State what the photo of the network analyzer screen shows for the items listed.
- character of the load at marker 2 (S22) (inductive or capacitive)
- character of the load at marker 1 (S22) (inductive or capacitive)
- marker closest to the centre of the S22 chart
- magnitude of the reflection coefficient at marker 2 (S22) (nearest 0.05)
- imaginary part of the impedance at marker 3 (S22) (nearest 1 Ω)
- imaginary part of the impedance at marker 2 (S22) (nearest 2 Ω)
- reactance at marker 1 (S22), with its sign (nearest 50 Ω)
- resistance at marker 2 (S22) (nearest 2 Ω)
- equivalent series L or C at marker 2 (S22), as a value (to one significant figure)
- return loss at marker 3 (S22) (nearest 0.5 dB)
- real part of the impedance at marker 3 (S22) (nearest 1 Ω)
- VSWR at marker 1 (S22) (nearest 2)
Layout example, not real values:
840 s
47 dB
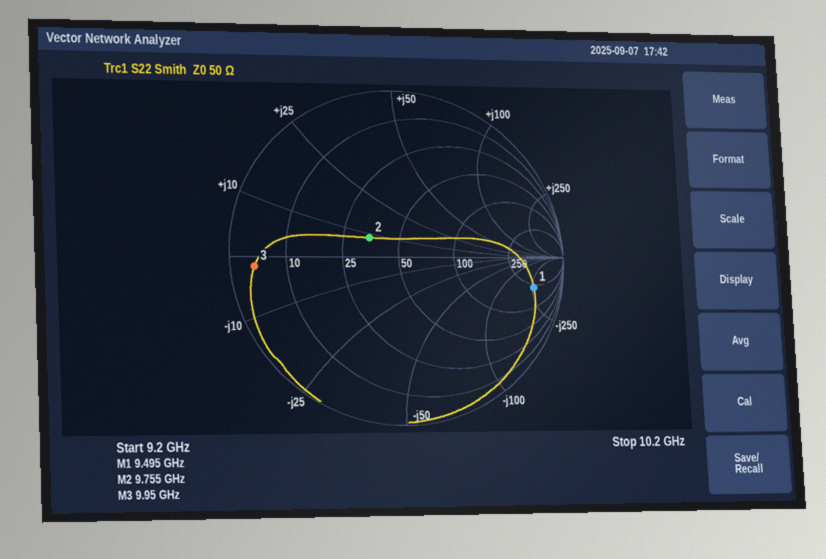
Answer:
inductive
capacitive
marker 2
0.20
-2 Ω
+8 Ω
-250 Ω
34 Ω
100 pH
1.5 dB
4 Ω
10
